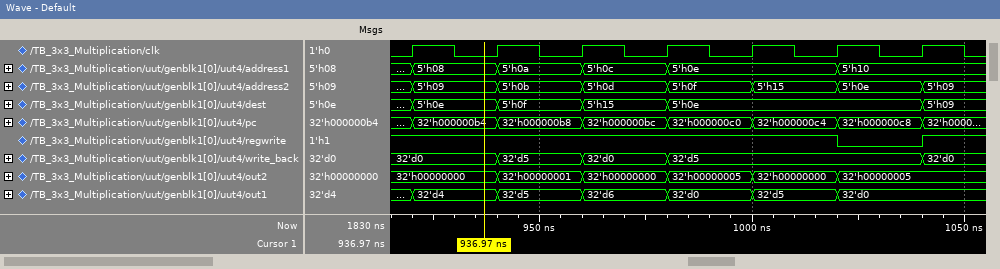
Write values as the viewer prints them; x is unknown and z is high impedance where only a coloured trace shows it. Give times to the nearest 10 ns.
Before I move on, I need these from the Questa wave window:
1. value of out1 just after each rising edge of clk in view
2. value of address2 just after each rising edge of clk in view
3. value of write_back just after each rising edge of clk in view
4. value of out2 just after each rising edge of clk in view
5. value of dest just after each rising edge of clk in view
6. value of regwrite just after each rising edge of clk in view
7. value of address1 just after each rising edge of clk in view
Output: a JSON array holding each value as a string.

["32'd4, 32'd5, 32'd6, 32'd0, 32'd5, 32'd0, 32'd0", "5'h09, 5'h0b, 5'h0d, 5'h0f, 5'h15, 5'h0e, 5'h09", "32'd0, 32'd5, 32'd0, 32'd5, 32'd5, 32'd5, 32'd0", "32'h00000000, 32'h00000001, 32'h00000000, 32'h00000005, 32'h00000000, 32'h00000005, 32'h00000005", "5'h0e, 5'h0f, 5'h15, 5'h0e, 5'h0e, 5'h0e, 5'h09", "1 1 1 1 1 0 1", "5'h08, 5'h0a, 5'h0c, 5'h0e, 5'h0e, 5'h10, 5'h10"]
